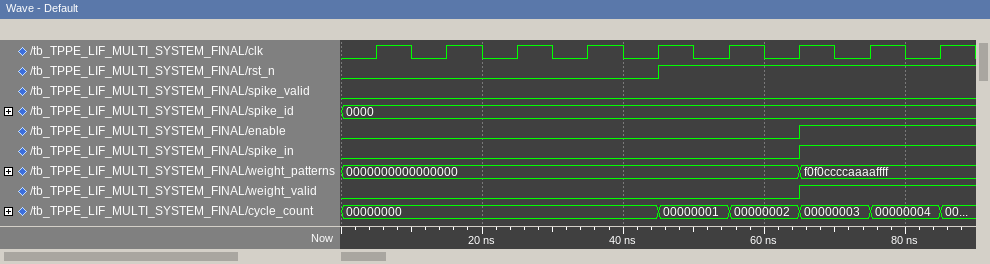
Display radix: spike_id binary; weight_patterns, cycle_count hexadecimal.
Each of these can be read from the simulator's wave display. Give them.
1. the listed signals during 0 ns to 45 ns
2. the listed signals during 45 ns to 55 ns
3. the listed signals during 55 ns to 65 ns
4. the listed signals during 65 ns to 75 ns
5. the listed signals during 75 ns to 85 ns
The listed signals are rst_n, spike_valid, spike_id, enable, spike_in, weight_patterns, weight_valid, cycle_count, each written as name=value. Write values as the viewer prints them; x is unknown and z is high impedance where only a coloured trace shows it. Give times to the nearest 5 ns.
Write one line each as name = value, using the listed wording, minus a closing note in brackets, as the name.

the listed signals during 0 ns to 45 ns = rst_n=0, spike_valid=0, spike_id=0000, enable=0, spike_in=0, weight_patterns=0000000000000000, weight_valid=0, cycle_count=00000000
the listed signals during 45 ns to 55 ns = rst_n=1, spike_valid=0, spike_id=0000, enable=0, spike_in=0, weight_patterns=0000000000000000, weight_valid=0, cycle_count=00000001
the listed signals during 55 ns to 65 ns = rst_n=1, spike_valid=0, spike_id=0000, enable=0, spike_in=0, weight_patterns=0000000000000000, weight_valid=0, cycle_count=00000002
the listed signals during 65 ns to 75 ns = rst_n=1, spike_valid=0, spike_id=0000, enable=1, spike_in=1, weight_patterns=f0f0ccccaaaaffff, weight_valid=1, cycle_count=00000003
the listed signals during 75 ns to 85 ns = rst_n=1, spike_valid=0, spike_id=0000, enable=1, spike_in=1, weight_patterns=f0f0ccccaaaaffff, weight_valid=1, cycle_count=00000004
